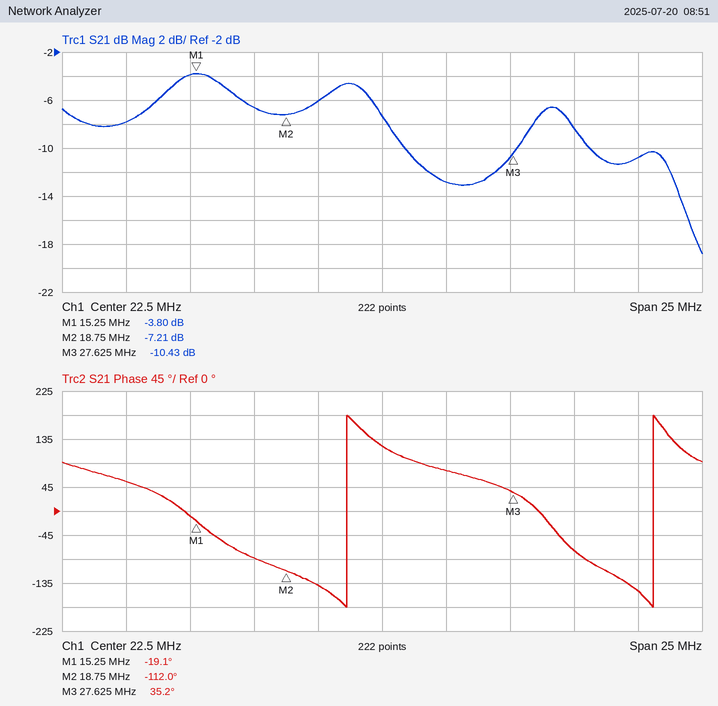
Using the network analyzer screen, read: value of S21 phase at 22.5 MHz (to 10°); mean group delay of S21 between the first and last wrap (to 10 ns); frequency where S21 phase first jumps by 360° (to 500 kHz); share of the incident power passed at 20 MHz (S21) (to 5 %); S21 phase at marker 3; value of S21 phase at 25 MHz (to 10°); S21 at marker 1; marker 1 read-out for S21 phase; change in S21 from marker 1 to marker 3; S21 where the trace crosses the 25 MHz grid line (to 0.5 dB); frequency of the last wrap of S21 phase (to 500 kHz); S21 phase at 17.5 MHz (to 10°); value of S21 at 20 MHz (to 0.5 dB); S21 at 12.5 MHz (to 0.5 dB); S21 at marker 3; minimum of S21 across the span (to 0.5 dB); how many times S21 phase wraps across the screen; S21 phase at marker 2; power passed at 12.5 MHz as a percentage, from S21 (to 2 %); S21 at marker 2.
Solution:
120°
80 ns
21.0 MHz
25 %
35.2°
80°
-3.80 dB
-19.1°
-6.63 dB
-13.0 dB
33.0 MHz
-90°
-6.0 dB
-8.0 dB
-10.43 dB
-19.0 dB
2
-112.0°
16 %
-7.21 dB
